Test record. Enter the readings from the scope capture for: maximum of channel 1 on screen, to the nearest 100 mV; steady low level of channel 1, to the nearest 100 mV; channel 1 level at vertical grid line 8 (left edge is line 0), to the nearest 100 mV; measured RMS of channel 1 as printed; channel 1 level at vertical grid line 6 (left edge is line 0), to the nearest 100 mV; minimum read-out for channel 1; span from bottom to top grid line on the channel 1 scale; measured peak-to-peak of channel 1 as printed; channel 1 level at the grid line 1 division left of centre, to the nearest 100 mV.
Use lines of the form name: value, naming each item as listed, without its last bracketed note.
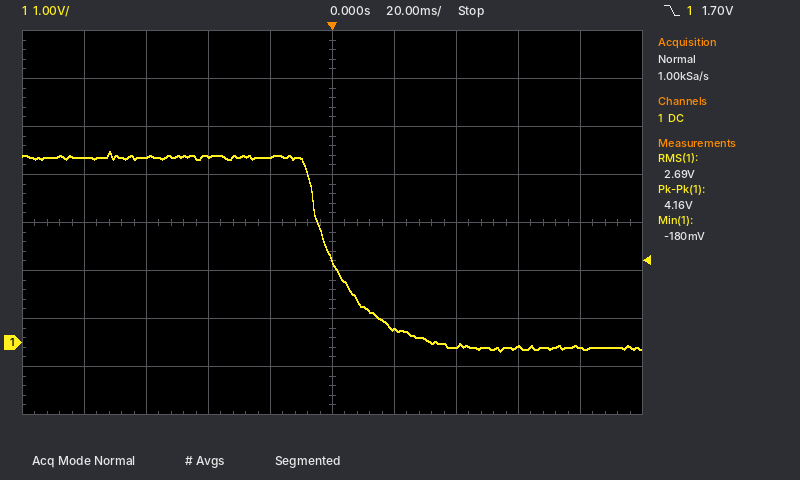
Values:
maximum of channel 1 on screen, to the nearest 100 mV: 4.0 V
steady low level of channel 1, to the nearest 100 mV: -100 mV
channel 1 level at vertical grid line 8 (left edge is line 0), to the nearest 100 mV: -100 mV
measured RMS of channel 1 as printed: 2.69 V
channel 1 level at vertical grid line 6 (left edge is line 0), to the nearest 100 mV: 300 mV
minimum read-out for channel 1: -180 mV
span from bottom to top grid line on the channel 1 scale: 8 V
measured peak-to-peak of channel 1 as printed: 4.16 V
channel 1 level at the grid line 1 division left of centre, to the nearest 100 mV: 3.9 V
